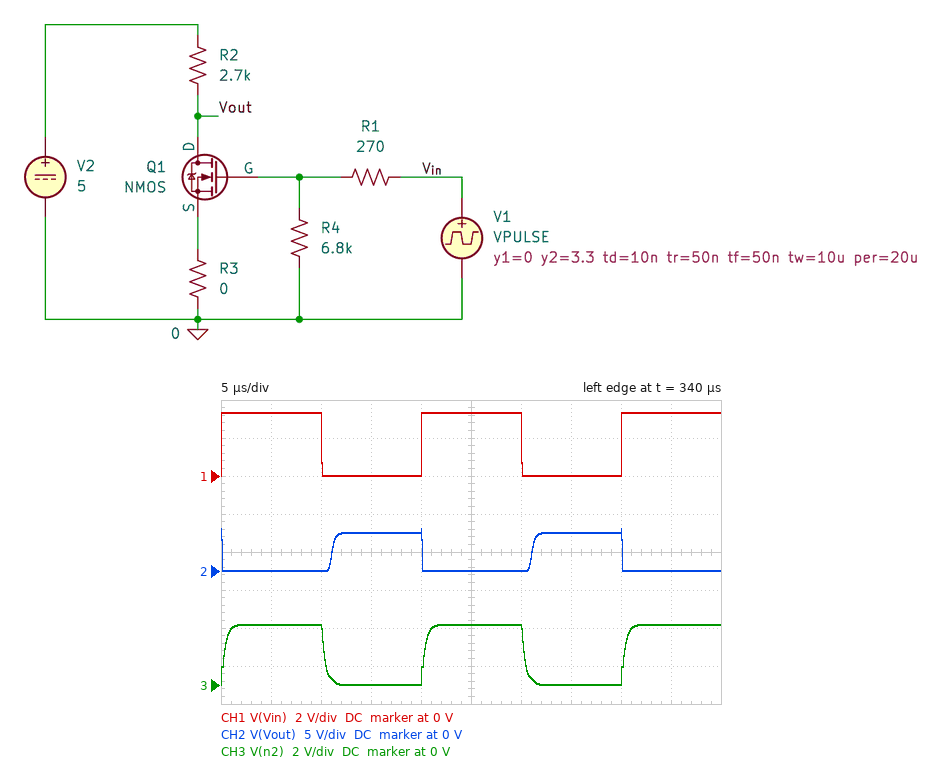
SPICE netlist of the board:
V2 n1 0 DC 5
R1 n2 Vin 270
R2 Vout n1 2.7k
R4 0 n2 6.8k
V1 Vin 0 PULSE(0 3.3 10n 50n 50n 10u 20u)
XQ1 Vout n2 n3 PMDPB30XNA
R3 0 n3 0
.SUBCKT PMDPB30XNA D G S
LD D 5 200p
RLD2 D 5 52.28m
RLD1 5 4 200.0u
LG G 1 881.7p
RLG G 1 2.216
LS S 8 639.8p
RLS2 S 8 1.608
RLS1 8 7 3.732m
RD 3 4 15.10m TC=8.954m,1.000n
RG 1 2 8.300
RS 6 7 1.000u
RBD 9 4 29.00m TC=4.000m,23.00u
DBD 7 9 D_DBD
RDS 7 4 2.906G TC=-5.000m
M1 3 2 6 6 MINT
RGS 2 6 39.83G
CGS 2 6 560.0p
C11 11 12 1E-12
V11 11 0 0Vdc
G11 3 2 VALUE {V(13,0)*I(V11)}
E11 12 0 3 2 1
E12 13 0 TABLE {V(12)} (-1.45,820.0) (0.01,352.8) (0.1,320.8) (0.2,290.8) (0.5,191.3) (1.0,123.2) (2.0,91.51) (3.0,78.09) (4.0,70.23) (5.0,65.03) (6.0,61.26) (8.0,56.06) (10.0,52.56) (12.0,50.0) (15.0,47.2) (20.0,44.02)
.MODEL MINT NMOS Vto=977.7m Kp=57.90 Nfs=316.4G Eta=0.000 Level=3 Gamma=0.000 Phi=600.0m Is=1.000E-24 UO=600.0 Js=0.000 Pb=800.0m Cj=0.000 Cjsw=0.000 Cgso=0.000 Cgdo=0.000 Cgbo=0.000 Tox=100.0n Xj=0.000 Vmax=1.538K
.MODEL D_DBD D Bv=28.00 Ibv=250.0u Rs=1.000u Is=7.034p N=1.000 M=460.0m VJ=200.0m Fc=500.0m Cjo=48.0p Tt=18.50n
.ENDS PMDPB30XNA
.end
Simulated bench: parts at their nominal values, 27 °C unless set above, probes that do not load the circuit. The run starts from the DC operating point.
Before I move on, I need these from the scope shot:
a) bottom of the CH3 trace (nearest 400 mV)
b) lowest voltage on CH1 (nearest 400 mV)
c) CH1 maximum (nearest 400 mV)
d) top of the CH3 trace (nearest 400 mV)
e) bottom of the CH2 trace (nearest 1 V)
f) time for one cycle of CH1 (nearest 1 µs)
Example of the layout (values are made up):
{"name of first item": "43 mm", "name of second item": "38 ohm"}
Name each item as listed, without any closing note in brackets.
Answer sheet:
{"bottom of the CH3 trace": "0 V", "lowest voltage on CH1": "0 V", "CH1 maximum": "3.2 V", "top of the CH3 trace": "3.2 V", "bottom of the CH2 trace": "0 V", "time for one cycle of CH1": "20 µs"}
